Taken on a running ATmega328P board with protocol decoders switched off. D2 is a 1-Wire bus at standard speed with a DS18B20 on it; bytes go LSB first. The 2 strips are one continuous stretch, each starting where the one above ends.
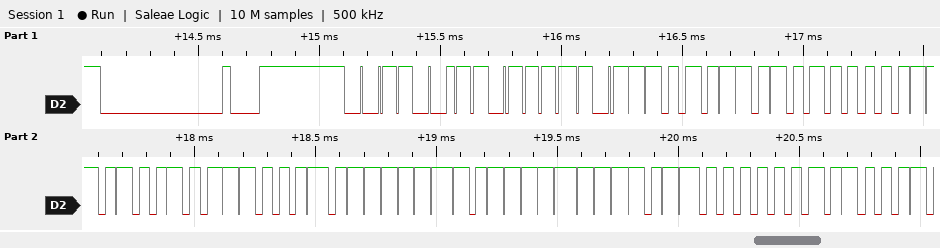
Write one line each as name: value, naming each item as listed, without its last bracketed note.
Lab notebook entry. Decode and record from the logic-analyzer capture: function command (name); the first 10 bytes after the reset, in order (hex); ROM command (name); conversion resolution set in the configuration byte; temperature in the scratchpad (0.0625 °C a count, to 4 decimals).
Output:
function command: Read Scratchpad
the first 10 bytes after the reset, in order: CC BE 63 01 4B 46 7F FF 0D 10
ROM command: Skip ROM
conversion resolution set in the configuration byte: 12 bits
temperature in the scratchpad: 22.1875 °C
